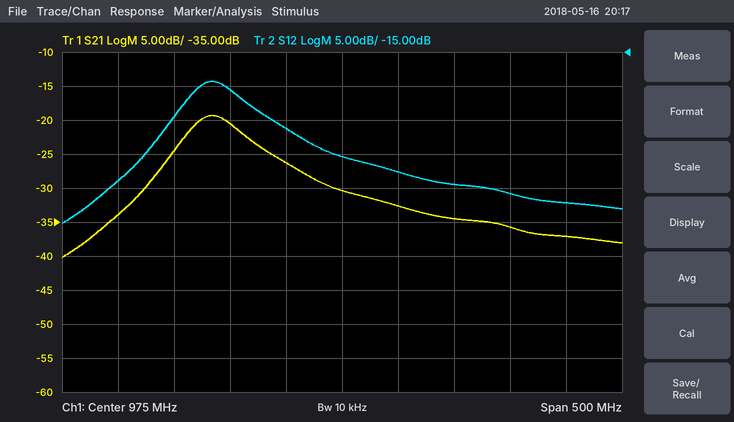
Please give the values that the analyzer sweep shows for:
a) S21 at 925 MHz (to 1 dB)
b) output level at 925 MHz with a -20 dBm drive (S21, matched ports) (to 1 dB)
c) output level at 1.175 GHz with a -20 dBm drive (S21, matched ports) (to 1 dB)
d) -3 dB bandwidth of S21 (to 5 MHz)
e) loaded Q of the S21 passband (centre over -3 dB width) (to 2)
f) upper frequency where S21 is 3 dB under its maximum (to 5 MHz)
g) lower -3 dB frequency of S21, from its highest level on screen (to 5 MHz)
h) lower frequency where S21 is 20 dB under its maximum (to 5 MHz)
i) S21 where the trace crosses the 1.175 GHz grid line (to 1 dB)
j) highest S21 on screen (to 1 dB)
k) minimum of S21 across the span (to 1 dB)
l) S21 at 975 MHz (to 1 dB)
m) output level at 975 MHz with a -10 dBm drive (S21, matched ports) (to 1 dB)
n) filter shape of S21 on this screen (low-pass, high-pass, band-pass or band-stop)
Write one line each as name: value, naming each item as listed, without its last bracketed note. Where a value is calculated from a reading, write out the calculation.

S21 at 925 MHz: -26 dB
output level at 925 MHz with a -20 dBm drive (S21, matched ports): -20 dBm + (-26 dB) = -46 dBm
output level at 1.175 GHz with a -20 dBm drive (S21, matched ports): -20 dBm + (-37 dB) = -57 dBm
-3 dB bandwidth of S21: 890 MHz − 835 MHz = 55 MHz
loaded Q of the S21 passband (centre over -3 dB width): 862.5 MHz / 55 MHz ≈ 16
upper frequency where S21 is 3 dB under its maximum: 890 MHz
lower -3 dB frequency of S21, from its highest level on screen: 835 MHz
lower frequency where S21 is 20 dB under its maximum: 735 MHz
S21 where the trace crosses the 1.175 GHz grid line: -37 dB
highest S21 on screen: -19 dB
minimum of S21 across the span: -40 dB
S21 at 975 MHz: -30 dB
output level at 975 MHz with a -10 dBm drive (S21, matched ports): -10 dBm + (-30 dB) = -40 dBm
filter shape of S21 on this screen: band-pass
